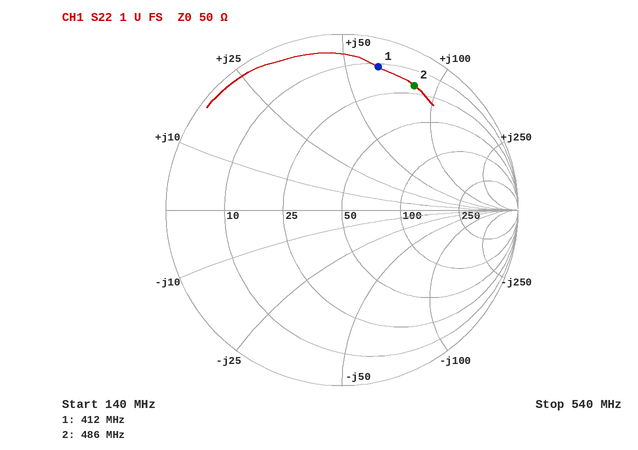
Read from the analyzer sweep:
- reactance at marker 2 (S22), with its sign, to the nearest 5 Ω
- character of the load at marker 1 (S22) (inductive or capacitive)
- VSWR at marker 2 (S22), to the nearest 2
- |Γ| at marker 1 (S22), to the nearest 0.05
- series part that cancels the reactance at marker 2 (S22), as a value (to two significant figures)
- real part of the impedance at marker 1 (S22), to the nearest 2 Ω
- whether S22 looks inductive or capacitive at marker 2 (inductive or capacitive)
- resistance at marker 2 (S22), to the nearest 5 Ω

+85 Ω
inductive
10
0.85
3.9 pF
12 Ω
inductive
20 Ω
